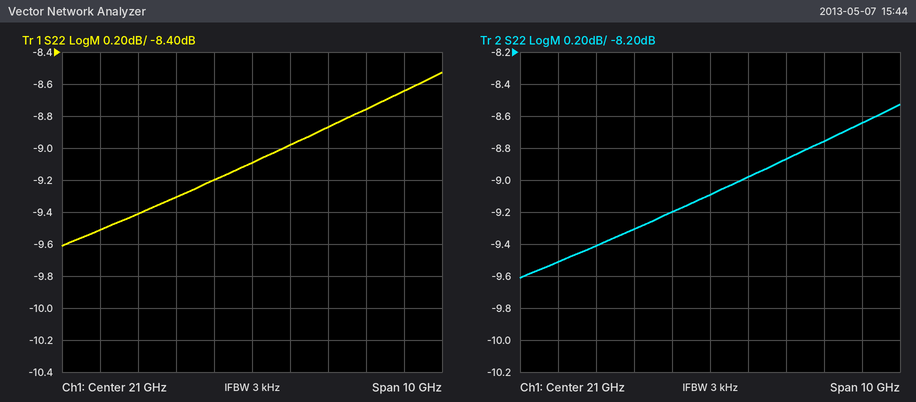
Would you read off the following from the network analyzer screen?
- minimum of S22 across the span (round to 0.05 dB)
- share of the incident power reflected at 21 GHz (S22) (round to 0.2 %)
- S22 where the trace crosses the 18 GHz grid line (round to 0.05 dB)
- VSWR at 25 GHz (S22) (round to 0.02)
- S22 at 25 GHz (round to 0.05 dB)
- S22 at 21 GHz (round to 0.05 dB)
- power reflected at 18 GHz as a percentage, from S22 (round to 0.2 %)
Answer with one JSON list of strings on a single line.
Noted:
["-9.60 dB", "12.4 %", "-9.40 dB", "2.18", "-8.65 dB", "-9.10 dB", "11.4 %"]
